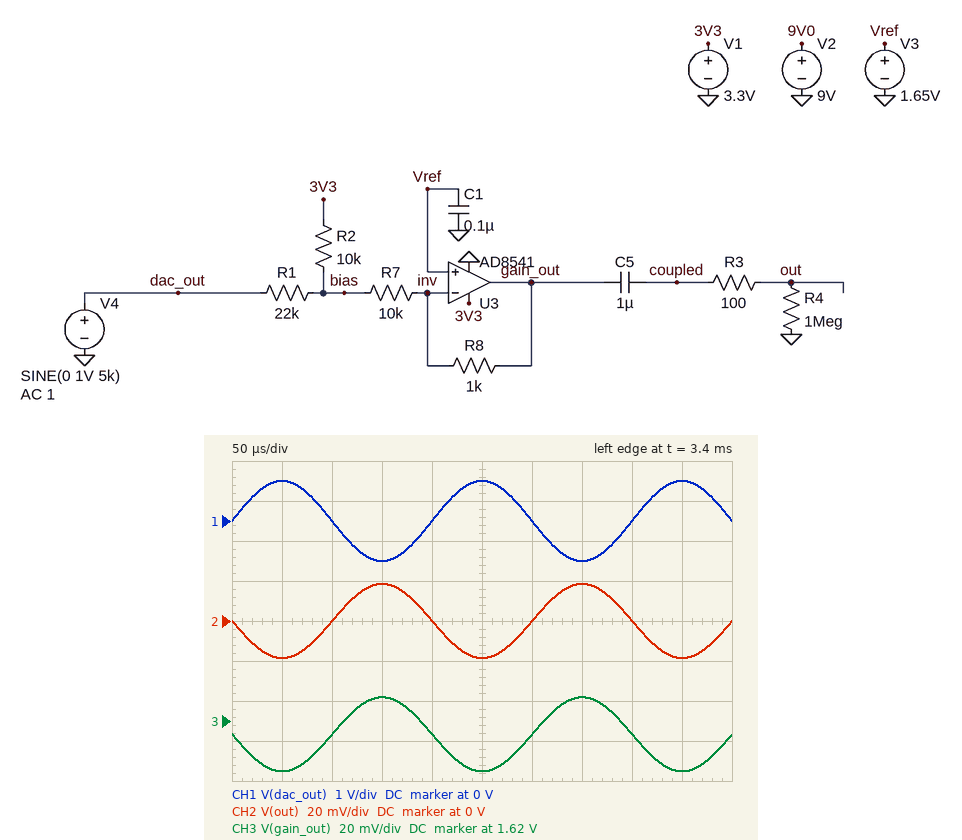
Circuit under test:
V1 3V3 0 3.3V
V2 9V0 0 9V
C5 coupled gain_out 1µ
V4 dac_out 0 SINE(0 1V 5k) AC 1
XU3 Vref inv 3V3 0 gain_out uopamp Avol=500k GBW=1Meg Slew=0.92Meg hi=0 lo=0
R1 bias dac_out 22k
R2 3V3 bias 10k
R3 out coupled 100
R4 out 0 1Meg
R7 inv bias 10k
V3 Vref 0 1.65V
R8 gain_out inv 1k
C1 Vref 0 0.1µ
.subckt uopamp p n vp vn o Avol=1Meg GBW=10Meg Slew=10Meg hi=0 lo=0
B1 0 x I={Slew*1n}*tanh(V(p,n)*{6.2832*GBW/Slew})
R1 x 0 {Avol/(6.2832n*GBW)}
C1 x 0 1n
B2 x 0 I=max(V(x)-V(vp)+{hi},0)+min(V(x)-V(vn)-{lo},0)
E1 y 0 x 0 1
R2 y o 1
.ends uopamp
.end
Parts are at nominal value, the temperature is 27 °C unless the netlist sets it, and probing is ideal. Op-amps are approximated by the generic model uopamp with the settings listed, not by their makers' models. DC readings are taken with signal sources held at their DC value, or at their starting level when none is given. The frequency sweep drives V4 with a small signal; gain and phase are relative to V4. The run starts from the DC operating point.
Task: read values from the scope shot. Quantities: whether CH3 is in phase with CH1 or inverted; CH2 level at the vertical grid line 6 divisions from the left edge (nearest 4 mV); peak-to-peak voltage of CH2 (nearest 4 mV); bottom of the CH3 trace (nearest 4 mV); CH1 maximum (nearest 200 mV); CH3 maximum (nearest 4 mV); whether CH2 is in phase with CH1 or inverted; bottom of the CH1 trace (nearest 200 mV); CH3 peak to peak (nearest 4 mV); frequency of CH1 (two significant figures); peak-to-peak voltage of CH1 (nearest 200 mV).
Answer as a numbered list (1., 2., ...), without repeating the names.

1. inverted
2. 0 V
3. 36 mV
4. 1.596 V
5. 1.0 V
6. 1.632 V
7. inverted
8. -1.0 V
9. 36 mV
10. 5.0 kHz
11. 2.0 V
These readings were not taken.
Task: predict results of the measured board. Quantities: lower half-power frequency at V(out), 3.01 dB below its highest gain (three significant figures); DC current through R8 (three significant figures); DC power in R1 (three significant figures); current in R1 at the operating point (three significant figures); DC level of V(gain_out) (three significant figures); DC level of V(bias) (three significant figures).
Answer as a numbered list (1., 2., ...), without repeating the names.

1. 159 mHz
2. 36.7 µA
3. 185 µW
4. 91.7 µA
5. 1.61 V
6. 2.02 V
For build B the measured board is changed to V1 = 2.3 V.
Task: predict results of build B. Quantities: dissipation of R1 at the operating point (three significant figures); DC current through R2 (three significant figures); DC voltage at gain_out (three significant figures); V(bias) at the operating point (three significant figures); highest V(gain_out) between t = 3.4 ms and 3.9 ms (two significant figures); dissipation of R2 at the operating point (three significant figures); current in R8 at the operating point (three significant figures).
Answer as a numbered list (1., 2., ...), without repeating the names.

1. 118 µW
2. 69.1 µA
3. 1.65 V
4. 1.61 V
5. 1.7 V
6. 47.7 µW
7. 4.07 µA
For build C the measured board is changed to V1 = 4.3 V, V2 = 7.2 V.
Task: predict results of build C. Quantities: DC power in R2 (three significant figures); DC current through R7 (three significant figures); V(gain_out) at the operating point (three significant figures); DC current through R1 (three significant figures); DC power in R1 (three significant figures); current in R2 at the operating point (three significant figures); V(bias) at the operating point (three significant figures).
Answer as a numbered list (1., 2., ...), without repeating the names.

1. 352 µW
2. 77.4 µA
3. 1.57 V
4. 110 µA
5. 267 µW
6. 188 µA
7. 2.42 V
